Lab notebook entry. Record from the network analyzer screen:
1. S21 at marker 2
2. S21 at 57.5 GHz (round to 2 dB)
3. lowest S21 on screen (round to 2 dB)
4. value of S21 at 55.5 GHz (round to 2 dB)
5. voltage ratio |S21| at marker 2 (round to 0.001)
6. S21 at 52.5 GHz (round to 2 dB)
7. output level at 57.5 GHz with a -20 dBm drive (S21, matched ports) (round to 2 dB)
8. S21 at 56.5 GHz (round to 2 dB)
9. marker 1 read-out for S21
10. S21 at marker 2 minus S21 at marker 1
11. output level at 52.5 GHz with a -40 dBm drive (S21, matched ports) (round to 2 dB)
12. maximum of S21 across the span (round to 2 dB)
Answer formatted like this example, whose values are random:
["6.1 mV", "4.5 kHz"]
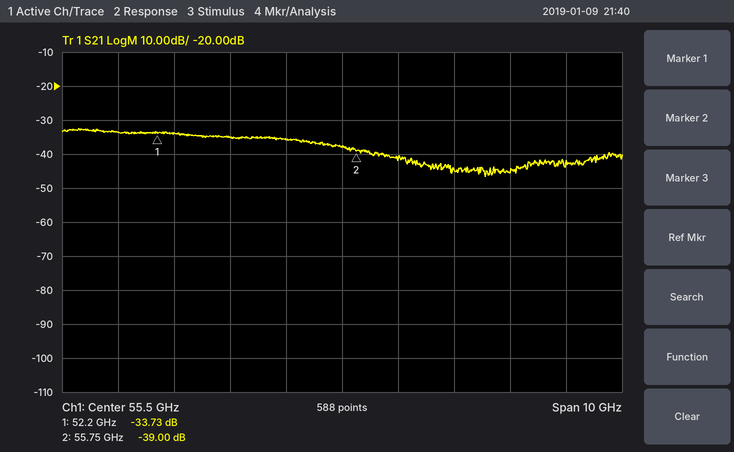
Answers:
["-39.00 dB", "-44 dB", "-46 dB", "-38 dB", "0.011", "-34 dB", "-64 dBm", "-42 dB", "-33.73 dB", "-5.27 dB", "-74 dBm", "-32 dB"]
